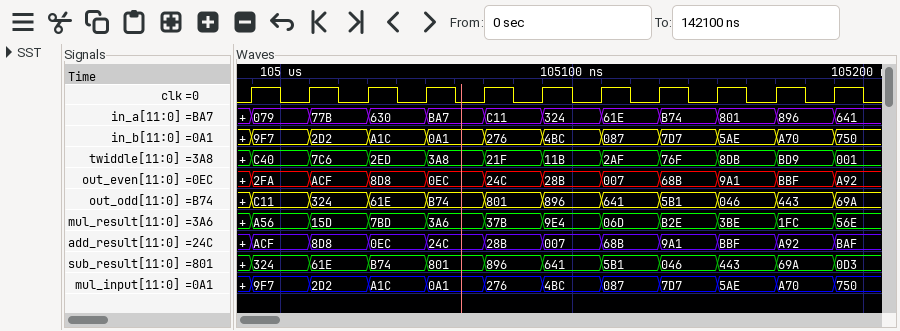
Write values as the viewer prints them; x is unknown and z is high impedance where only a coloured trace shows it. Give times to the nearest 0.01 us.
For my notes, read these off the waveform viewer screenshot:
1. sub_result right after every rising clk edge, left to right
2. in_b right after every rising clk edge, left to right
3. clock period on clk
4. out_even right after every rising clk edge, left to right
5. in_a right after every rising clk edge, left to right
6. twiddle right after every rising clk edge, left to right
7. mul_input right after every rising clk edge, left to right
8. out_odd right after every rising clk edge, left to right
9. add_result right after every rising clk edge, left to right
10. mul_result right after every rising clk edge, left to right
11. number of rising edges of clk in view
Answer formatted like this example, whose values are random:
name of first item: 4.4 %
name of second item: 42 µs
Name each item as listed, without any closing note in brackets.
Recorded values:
sub_result right after every rising clk edge, left to right: 324, 61E, B74, 801, 896, 641, 5B1, 046, 443, 69A, 0D3
in_b right after every rising clk edge, left to right: 9F7, 2D2, A1C, 0A1, 276, 4BC, 087, 7D7, 5AE, A70, 750
clock period on clk: 0.02 us
out_even right after every rising clk edge, left to right: 2FA, ACF, 8D8, 0EC, 24C, 28B, 007, 68B, 9A1, BBF, A92
in_a right after every rising clk edge, left to right: 079, 77B, 630, BA7, C11, 324, 61E, B74, 801, 896, 641
twiddle right after every rising clk edge, left to right: C40, 7C6, 2ED, 3A8, 21F, 11B, 2AF, 76F, 8DB, BD9, 001
mul_input right after every rising clk edge, left to right: 9F7, 2D2, A1C, 0A1, 276, 4BC, 087, 7D7, 5AE, A70, 750
out_odd right after every rising clk edge, left to right: C11, 324, 61E, B74, 801, 896, 641, 5B1, 046, 443, 69A
add_result right after every rising clk edge, left to right: ACF, 8D8, 0EC, 24C, 28B, 007, 68B, 9A1, BBF, A92, BAF
mul_result right after every rising clk edge, left to right: A56, 15D, 7BD, 3A6, 37B, 9E4, 06D, B2E, 3BE, 1FC, 56E
number of rising edges of clk in view: 11
